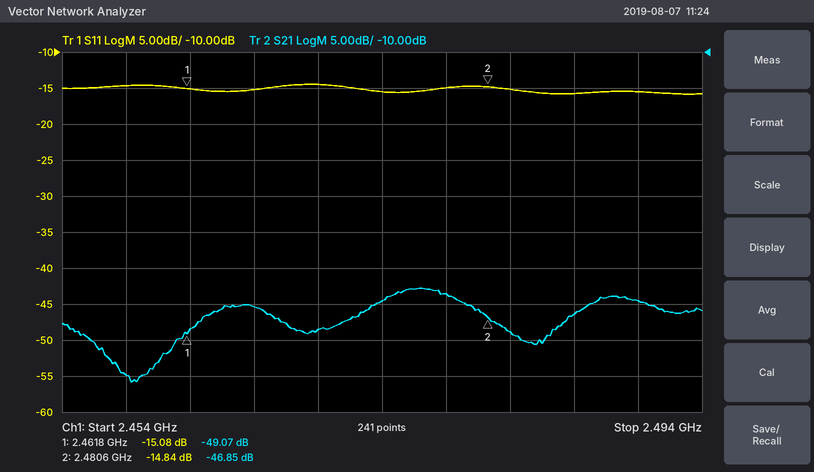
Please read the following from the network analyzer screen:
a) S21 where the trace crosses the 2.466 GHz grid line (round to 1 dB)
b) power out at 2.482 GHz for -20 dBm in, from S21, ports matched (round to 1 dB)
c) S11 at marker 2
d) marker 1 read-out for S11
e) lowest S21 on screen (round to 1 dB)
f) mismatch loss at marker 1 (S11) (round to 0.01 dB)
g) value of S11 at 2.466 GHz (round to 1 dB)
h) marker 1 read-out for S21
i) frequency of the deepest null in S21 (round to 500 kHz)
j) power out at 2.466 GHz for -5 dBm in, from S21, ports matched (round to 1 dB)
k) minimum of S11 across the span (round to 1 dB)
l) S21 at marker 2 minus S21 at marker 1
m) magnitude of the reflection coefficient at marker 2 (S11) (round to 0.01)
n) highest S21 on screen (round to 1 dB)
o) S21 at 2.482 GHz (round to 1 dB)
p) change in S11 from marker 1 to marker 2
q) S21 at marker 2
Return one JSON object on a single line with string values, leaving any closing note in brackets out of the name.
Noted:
{"S21 where the trace crosses the 2.466 GHz grid line": "-45 dB", "power out at 2.482 GHz for -20 dBm in, from S21, ports matched": "-69 dBm", "S11 at marker 2": "-14.84 dB", "marker 1 read-out for S11": "-15.08 dB", "lowest S21 on screen": "-56 dB", "mismatch loss at marker 1 (S11)": "0.14 dB", "value of S11 at 2.466 GHz": "-15 dB", "marker 1 read-out for S21": "-49.07 dB", "frequency of the deepest null in S21": "2.4585 GHz", "power out at 2.466 GHz for -5 dBm in, from S21, ports matched": "-50 dBm", "minimum of S11 across the span": "-16 dB", "S21 at marker 2 minus S21 at marker 1": "2.22 dB", "magnitude of the reflection coefficient at marker 2 (S11)": "0.18", "highest S21 on screen": "-43 dB", "S21 at 2.482 GHz": "-49 dB", "change in S11 from marker 1 to marker 2": "0.24 dB", "S21 at marker 2": "-46.85 dB"}
